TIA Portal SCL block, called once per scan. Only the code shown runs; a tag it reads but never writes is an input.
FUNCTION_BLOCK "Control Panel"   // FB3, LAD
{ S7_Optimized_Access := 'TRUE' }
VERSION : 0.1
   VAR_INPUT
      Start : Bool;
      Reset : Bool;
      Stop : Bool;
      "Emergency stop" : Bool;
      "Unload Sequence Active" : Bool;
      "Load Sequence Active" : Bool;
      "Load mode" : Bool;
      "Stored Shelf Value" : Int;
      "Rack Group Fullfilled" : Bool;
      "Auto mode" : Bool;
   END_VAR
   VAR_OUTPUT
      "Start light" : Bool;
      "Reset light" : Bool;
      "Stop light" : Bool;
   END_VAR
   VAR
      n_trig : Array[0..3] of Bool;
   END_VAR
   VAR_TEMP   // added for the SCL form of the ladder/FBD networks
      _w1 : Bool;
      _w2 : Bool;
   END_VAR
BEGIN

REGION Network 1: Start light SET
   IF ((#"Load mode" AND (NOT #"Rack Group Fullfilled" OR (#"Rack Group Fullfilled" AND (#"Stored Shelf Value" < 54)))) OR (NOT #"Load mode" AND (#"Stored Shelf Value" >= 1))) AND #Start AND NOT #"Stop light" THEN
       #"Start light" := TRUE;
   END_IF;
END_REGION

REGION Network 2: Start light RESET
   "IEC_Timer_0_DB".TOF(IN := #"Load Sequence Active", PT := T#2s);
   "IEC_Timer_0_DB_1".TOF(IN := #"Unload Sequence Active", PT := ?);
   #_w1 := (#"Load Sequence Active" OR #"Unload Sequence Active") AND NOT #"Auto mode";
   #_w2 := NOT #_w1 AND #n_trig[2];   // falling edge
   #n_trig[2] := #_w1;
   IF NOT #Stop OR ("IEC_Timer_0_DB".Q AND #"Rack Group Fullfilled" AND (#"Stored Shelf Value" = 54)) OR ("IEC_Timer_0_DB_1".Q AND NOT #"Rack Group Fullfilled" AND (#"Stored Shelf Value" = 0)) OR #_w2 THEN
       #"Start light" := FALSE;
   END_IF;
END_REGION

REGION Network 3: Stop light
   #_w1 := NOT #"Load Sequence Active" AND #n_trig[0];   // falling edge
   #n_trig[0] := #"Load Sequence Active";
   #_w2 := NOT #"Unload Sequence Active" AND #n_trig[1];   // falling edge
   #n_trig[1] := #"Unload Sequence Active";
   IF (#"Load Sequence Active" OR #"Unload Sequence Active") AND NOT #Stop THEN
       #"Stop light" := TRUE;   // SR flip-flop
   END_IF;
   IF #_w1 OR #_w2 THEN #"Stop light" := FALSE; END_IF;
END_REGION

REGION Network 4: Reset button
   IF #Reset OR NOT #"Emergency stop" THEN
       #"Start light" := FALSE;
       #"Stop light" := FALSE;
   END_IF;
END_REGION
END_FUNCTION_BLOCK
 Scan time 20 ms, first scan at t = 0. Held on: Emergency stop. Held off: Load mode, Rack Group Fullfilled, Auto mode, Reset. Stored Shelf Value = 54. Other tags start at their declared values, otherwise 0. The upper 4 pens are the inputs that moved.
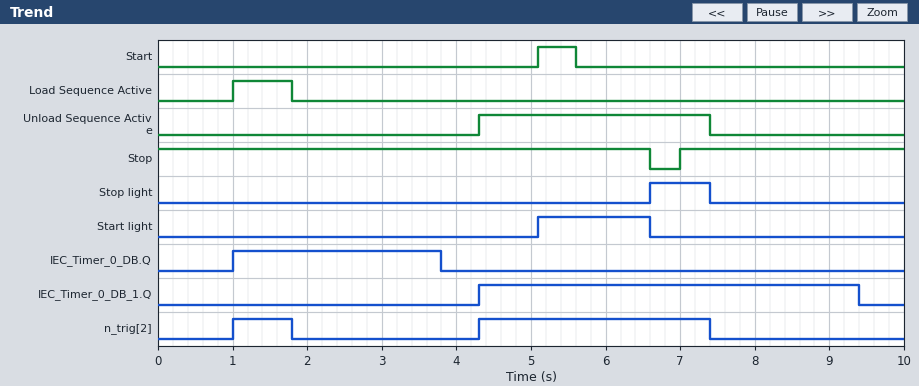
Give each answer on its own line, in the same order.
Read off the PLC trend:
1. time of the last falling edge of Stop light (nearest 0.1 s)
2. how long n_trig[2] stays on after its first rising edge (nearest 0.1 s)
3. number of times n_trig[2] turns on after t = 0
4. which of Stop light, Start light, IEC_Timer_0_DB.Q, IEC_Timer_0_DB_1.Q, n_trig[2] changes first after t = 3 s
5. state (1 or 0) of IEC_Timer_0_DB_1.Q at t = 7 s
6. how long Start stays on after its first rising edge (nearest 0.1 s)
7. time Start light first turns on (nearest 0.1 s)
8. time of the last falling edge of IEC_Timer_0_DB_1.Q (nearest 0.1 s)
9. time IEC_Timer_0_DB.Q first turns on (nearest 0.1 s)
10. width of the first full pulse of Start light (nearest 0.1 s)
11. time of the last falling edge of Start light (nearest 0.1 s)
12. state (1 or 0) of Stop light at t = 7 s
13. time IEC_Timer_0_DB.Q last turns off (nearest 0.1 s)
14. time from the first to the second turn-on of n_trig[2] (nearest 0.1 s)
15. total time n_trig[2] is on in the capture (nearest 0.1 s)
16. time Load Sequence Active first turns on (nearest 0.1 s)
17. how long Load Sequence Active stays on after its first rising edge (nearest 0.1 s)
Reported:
7.4 s
0.8 s
2
IEC_Timer_0_DB.Q
1
0.5 s
5.1 s
9.4 s
1.0 s
1.5 s
6.6 s
1
3.8 s
3.3 s
3.9 s
1.0 s
0.8 s
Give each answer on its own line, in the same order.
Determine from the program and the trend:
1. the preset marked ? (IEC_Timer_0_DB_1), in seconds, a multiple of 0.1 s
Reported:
2.0 s
